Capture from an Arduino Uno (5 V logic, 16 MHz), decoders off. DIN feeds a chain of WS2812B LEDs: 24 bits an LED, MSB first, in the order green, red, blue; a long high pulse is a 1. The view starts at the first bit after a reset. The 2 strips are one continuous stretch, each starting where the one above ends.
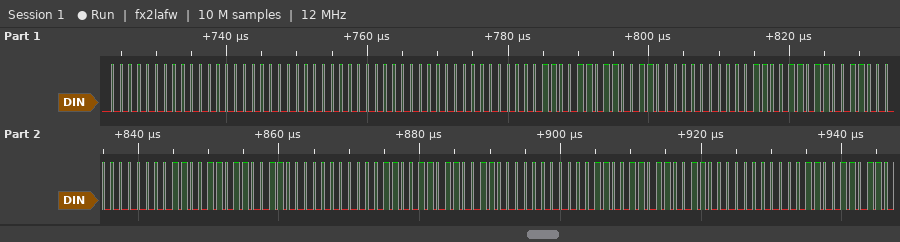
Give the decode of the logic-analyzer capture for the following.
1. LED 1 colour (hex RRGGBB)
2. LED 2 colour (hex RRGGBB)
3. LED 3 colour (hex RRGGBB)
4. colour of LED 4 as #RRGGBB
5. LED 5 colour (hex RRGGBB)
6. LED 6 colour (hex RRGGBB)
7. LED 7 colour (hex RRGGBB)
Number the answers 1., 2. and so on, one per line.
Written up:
1. #000000
2. #000000
3. #CC6600
4. #CC6600
5. #CC6600
6. #CC6600
7. #CC6600
